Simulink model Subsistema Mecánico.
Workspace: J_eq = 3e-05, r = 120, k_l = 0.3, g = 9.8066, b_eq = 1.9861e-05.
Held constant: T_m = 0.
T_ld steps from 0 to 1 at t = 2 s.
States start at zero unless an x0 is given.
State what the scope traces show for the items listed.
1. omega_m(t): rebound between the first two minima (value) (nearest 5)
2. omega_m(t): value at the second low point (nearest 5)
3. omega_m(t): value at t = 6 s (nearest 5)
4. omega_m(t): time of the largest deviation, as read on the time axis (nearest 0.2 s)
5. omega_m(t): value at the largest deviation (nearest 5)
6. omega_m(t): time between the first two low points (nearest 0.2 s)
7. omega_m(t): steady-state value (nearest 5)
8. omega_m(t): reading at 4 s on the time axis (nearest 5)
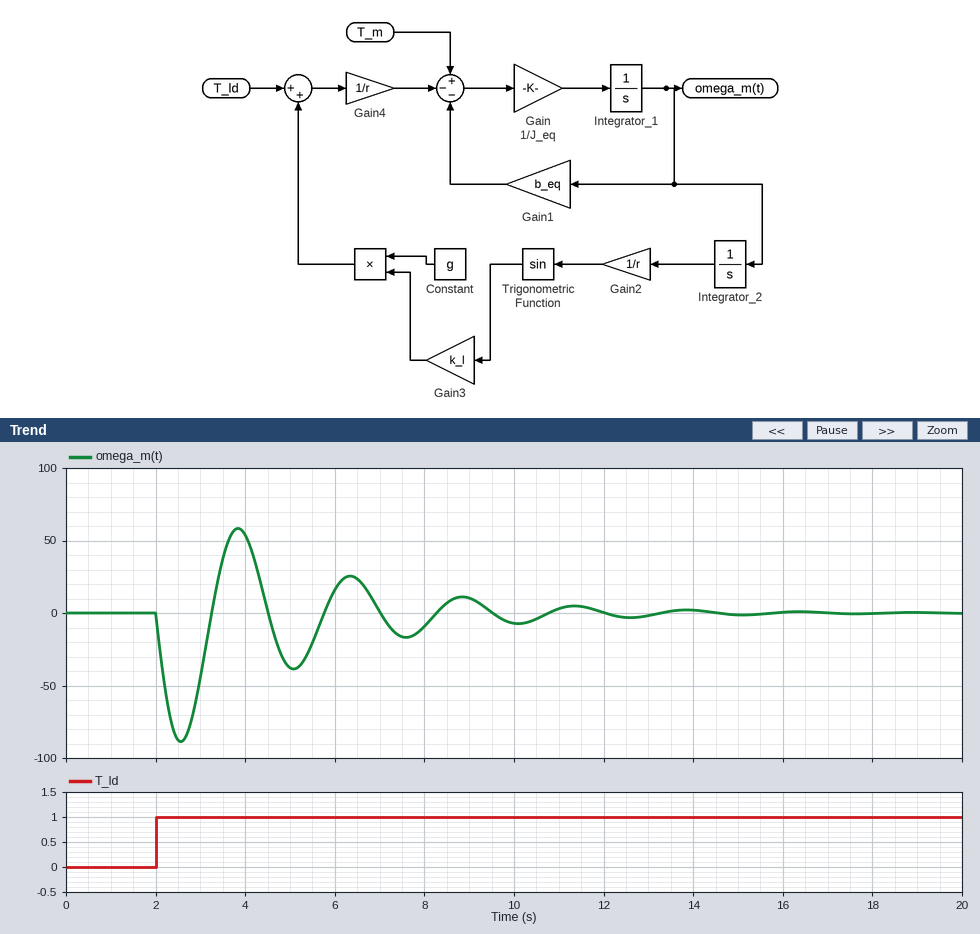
60
-40
15
2.6 s
-90
2.6 s
0
55
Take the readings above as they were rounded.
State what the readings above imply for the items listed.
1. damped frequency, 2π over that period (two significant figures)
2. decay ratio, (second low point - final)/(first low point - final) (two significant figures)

2.4 rad/s
0.44
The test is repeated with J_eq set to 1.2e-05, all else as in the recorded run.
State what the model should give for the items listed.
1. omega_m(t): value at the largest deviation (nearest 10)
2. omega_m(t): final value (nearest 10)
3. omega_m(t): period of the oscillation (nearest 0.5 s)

-130
0
1.5 s
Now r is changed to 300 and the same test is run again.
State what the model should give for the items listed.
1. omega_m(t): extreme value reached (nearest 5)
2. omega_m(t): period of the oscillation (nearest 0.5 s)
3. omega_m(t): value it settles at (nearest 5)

-70
6.5 s
0
